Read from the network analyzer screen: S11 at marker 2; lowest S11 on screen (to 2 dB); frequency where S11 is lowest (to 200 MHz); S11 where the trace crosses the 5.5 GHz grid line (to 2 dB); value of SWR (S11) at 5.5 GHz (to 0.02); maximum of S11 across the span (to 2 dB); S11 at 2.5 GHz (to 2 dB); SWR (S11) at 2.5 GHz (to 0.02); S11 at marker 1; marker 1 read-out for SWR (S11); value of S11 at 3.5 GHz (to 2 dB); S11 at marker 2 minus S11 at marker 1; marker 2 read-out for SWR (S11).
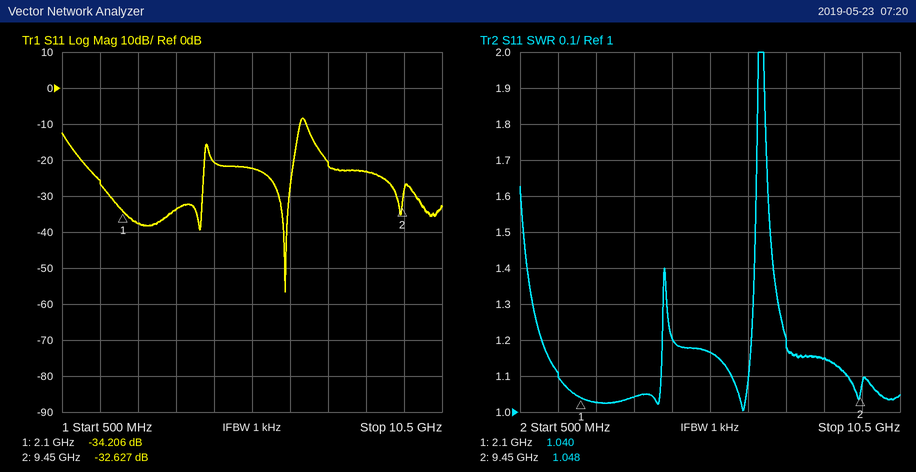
-32.627 dB
-56 dB
6.4 GHz
-22 dB
1.16
-8 dB
-38 dB
1.02
-34.206 dB
1.040
-34 dB
1.579 dB
1.048
